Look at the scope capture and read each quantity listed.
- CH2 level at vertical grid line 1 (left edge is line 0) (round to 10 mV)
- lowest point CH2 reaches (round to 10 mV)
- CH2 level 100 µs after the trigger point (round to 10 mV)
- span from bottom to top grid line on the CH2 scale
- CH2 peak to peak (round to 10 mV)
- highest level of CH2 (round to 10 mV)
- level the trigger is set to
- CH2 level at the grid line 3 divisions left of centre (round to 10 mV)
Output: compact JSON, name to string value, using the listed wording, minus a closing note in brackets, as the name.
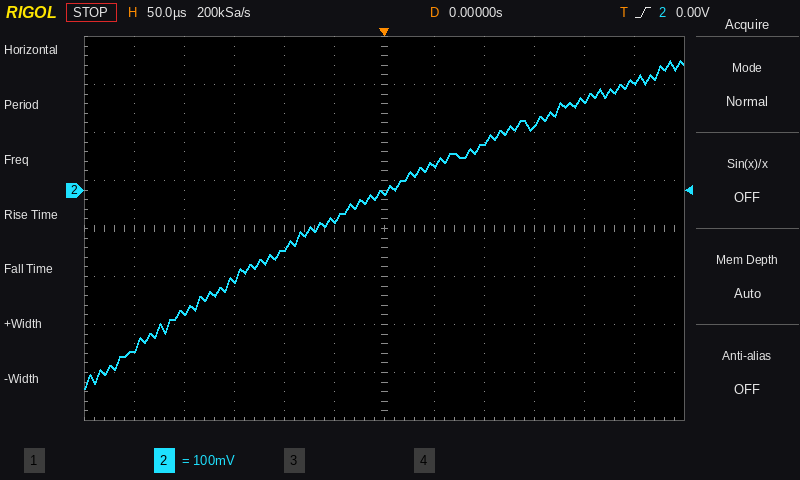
{"CH2 level at vertical grid line 1 (left edge is line 0)": "-330 mV", "lowest point CH2 reaches": "-410 mV", "CH2 level 100 µs after the trigger point": "100 mV", "span from bottom to top grid line on the CH2 scale": "800 mV", "CH2 peak to peak": "680 mV", "highest level of CH2": "270 mV", "level the trigger is set to": "0.00 V", "CH2 level at the grid line 3 divisions left of centre": "-190 mV"}
